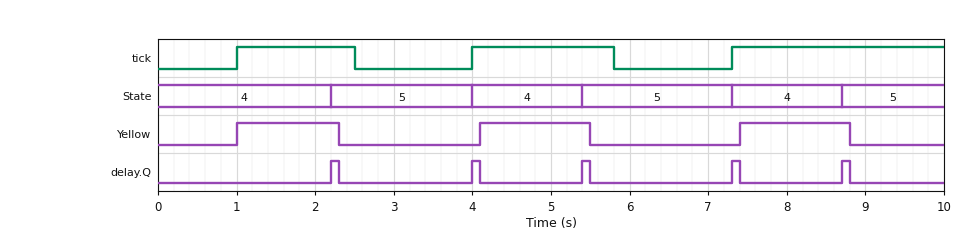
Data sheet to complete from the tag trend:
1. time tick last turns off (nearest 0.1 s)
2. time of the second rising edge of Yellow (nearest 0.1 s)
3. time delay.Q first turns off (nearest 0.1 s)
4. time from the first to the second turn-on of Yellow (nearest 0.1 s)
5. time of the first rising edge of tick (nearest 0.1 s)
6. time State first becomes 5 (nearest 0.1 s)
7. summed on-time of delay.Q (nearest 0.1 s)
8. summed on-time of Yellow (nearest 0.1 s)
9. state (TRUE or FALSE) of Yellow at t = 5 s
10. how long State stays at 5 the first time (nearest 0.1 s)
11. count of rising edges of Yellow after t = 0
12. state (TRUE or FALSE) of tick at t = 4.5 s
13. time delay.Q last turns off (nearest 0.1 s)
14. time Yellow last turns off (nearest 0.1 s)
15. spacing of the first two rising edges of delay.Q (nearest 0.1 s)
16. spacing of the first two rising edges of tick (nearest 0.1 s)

5.8 s
4.1 s
2.3 s
3.1 s
1.0 s
2.2 s
0.5 s
4.1 s
TRUE
1.8 s
3
TRUE
8.8 s
8.8 s
1.8 s
3.0 s
